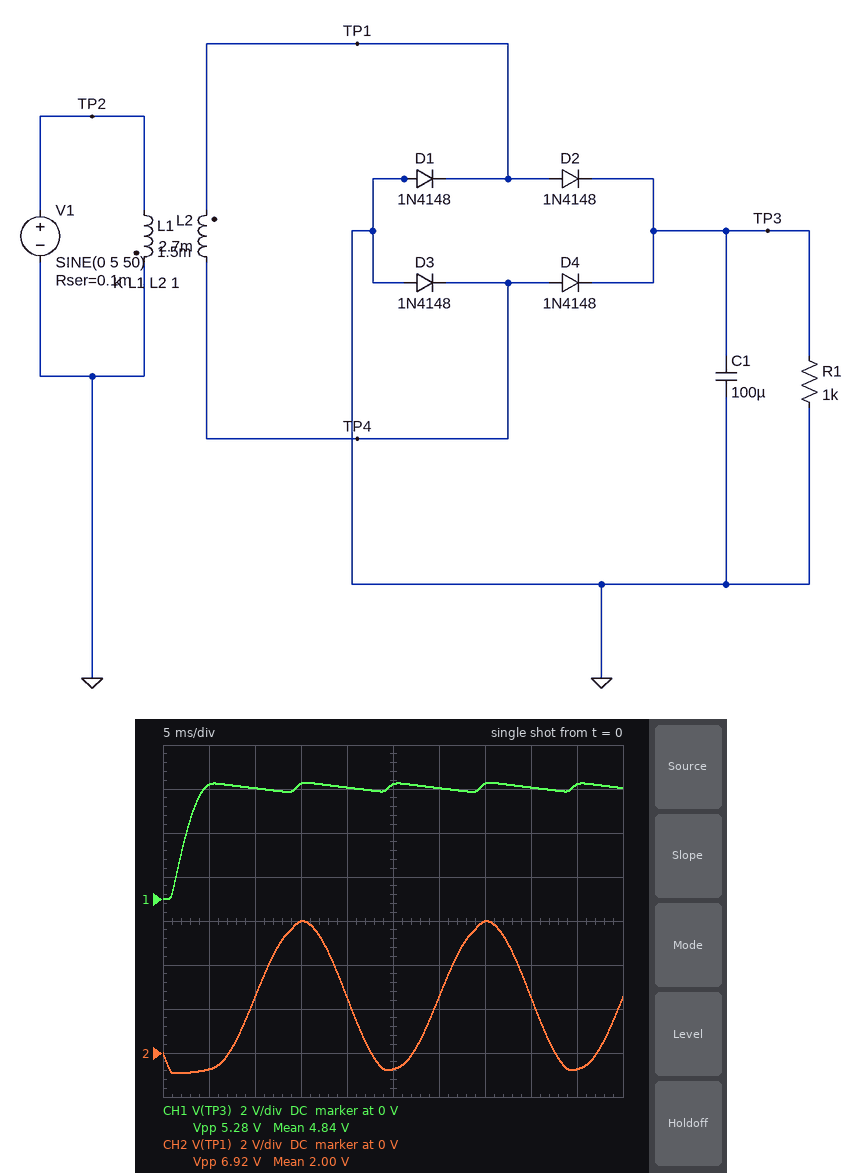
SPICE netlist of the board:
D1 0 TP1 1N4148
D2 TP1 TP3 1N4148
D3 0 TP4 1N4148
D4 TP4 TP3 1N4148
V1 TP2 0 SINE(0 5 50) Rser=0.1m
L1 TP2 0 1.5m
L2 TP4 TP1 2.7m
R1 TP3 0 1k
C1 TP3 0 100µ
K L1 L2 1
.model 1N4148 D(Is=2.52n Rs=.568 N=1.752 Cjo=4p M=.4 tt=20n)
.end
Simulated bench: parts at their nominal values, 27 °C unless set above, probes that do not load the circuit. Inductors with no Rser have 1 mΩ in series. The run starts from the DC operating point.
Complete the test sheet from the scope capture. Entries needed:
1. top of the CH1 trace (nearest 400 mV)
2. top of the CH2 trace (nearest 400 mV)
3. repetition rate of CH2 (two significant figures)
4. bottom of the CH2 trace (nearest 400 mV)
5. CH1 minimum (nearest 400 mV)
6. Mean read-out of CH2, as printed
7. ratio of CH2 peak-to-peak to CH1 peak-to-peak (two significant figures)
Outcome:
5.2 V
6.0 V
50 Hz
-800 mV
0 V
2.00 V
1.3
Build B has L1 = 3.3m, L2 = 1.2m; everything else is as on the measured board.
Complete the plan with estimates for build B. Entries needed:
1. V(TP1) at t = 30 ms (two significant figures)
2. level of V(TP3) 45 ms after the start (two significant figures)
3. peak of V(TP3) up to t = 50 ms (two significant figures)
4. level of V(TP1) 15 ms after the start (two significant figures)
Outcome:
800 mV
1.6 V
1.7 V
2.3 V
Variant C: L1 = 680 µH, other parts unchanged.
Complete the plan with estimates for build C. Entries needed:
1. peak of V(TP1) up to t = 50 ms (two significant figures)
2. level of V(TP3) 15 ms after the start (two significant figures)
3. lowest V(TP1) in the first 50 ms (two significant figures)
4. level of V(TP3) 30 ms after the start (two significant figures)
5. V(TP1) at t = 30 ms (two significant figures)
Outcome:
9.3 V
8.5 V
-1.0 V
8.1 V
4.1 V
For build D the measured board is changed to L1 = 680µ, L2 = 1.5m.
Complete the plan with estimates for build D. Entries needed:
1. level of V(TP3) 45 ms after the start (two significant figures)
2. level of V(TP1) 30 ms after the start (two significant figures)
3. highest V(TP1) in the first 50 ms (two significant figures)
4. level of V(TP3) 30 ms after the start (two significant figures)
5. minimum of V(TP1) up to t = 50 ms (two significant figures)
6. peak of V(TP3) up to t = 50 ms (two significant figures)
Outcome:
5.9 V
2.9 V
6.7 V
5.7 V
-950 mV
6.0 V
